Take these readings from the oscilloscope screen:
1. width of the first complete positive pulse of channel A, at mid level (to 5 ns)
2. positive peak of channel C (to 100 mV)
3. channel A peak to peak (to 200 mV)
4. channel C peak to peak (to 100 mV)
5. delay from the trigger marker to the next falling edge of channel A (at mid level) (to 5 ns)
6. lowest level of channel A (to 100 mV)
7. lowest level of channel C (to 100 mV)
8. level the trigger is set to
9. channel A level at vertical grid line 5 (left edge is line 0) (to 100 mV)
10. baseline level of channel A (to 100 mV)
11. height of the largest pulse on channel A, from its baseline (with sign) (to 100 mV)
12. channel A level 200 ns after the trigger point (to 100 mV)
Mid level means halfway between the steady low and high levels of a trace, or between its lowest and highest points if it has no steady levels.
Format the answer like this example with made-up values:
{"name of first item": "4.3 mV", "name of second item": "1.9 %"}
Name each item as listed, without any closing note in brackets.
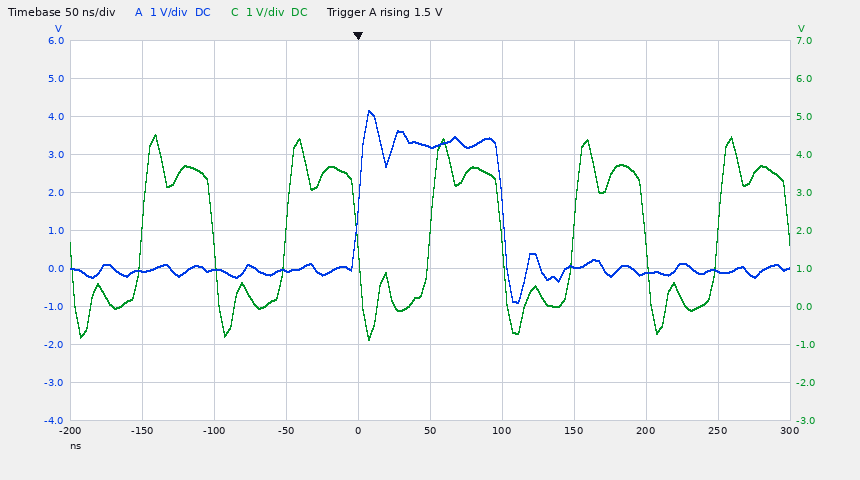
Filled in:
{"width of the first complete positive pulse of channel A, at mid level": "100 ns", "positive peak of channel C": "4.5 V", "channel A peak to peak": "5.0 V", "channel C peak to peak": "5.4 V", "delay from the trigger marker to the next falling edge of channel A (at mid level)": "100 ns", "lowest level of channel A": "-900 mV", "lowest level of channel C": "-900 mV", "level the trigger is set to": "1.5 V", "channel A level at vertical grid line 5 (left edge is line 0)": "3.2 V", "baseline level of channel A": "0.0 V", "height of the largest pulse on channel A, from its baseline (with sign)": "+4.2 V", "channel A level 200 ns after the trigger point": "-100 mV"}
